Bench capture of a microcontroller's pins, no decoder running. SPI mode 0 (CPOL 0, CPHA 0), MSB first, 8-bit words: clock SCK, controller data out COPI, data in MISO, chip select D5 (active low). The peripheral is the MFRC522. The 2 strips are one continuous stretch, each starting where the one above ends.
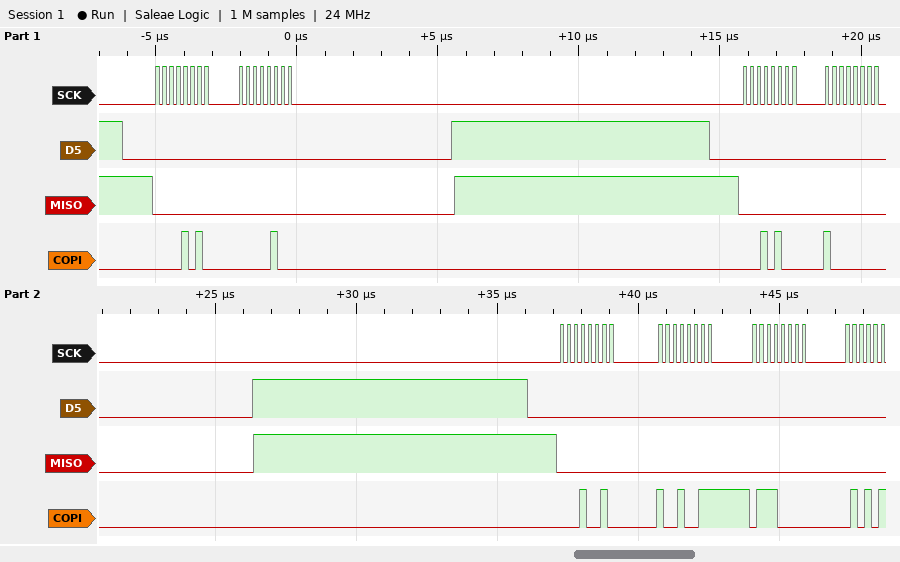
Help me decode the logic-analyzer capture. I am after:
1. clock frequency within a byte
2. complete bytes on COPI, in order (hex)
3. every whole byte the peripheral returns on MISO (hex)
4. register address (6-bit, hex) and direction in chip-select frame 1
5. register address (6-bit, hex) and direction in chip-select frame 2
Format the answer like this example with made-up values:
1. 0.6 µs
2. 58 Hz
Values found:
1. 4 MHz
2. 0A 04 14 80 12 93 70
3. 00 00 00 00 00 00 00
4. 0x05 write
5. 0x0A write
